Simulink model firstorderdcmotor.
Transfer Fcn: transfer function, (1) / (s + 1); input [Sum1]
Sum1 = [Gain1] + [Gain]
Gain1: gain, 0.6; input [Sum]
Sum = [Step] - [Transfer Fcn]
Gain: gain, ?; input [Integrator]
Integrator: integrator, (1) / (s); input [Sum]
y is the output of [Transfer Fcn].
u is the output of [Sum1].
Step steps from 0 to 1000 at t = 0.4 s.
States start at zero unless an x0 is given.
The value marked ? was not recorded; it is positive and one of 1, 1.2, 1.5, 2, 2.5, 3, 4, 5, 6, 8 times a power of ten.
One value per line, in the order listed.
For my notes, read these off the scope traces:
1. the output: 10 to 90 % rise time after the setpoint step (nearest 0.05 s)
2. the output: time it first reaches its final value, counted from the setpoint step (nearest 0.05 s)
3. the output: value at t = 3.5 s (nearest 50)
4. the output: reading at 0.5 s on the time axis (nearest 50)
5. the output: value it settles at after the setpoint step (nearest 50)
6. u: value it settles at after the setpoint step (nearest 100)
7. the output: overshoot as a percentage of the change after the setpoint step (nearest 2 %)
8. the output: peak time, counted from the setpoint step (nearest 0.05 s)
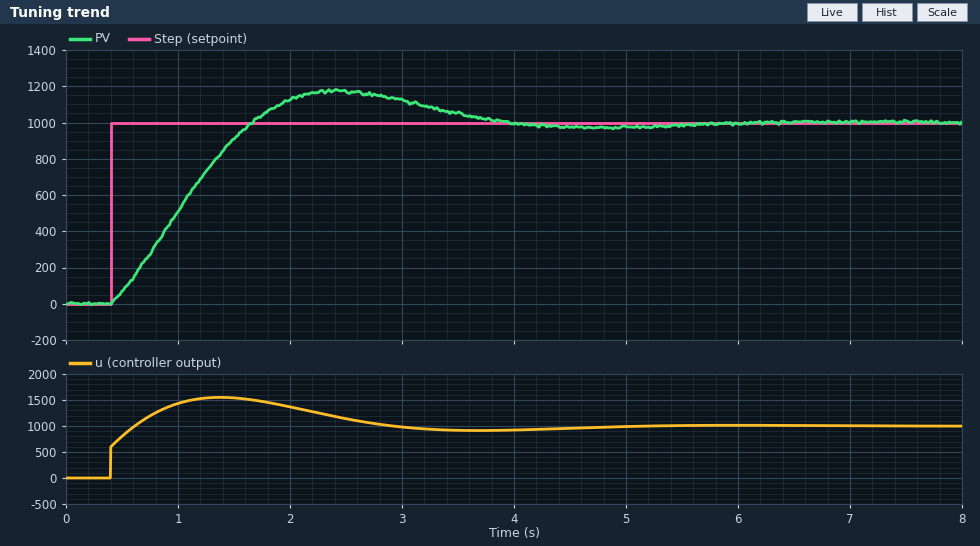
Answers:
0.95 s
1.25 s
1050
50
1000
1000
18 %
2.00 s
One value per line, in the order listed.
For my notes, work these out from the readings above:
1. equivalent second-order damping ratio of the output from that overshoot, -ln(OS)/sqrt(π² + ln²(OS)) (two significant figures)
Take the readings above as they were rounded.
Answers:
0.48
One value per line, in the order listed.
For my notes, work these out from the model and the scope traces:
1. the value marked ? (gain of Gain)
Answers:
2.5
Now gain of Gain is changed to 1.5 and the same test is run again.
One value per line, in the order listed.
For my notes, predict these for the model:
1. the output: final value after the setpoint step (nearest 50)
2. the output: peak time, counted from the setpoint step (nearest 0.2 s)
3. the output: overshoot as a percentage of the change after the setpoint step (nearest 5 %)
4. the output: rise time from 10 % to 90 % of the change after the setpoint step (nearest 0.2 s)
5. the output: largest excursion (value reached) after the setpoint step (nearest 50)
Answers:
1000
2.8 s
10 %
1.4 s
1100
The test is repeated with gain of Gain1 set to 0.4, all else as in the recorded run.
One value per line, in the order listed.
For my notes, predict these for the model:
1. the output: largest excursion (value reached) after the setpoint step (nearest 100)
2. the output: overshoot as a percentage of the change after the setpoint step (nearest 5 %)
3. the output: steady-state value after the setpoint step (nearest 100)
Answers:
1200
20 %
1000
